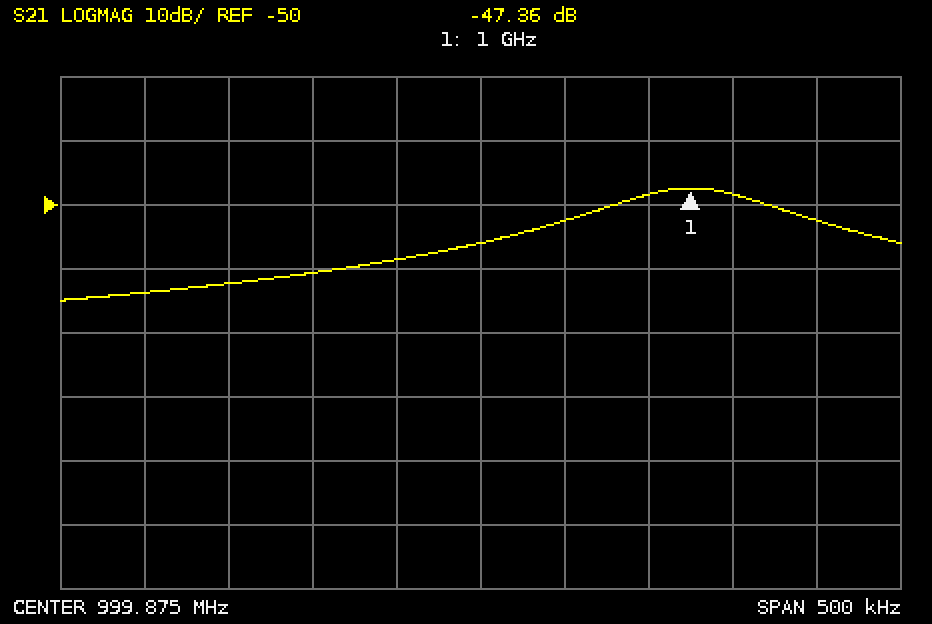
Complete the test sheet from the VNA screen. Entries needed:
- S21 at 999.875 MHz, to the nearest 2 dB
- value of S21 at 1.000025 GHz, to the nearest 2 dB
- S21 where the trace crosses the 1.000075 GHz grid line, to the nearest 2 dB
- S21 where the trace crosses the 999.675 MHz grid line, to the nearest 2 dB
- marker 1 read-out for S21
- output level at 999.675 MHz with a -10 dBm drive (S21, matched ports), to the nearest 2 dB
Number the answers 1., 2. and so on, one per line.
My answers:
1. -56 dB
2. -48 dB
3. -52 dB
4. -64 dB
5. -47.36 dB
6. -74 dBm
